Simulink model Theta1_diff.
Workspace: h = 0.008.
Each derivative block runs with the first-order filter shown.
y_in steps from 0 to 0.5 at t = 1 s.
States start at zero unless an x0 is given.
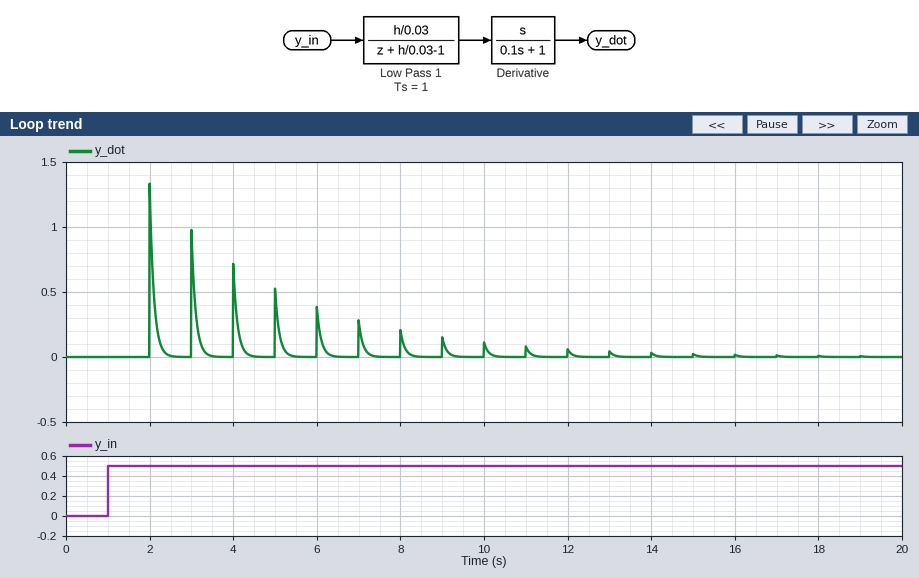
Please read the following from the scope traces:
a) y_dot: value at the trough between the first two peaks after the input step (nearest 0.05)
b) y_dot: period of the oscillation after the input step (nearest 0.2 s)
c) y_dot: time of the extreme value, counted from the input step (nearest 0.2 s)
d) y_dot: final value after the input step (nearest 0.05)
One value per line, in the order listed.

0.00
1.0 s
1.0 s
0.00
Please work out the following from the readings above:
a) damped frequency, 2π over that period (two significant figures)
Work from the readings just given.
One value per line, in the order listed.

6.3 rad/s
